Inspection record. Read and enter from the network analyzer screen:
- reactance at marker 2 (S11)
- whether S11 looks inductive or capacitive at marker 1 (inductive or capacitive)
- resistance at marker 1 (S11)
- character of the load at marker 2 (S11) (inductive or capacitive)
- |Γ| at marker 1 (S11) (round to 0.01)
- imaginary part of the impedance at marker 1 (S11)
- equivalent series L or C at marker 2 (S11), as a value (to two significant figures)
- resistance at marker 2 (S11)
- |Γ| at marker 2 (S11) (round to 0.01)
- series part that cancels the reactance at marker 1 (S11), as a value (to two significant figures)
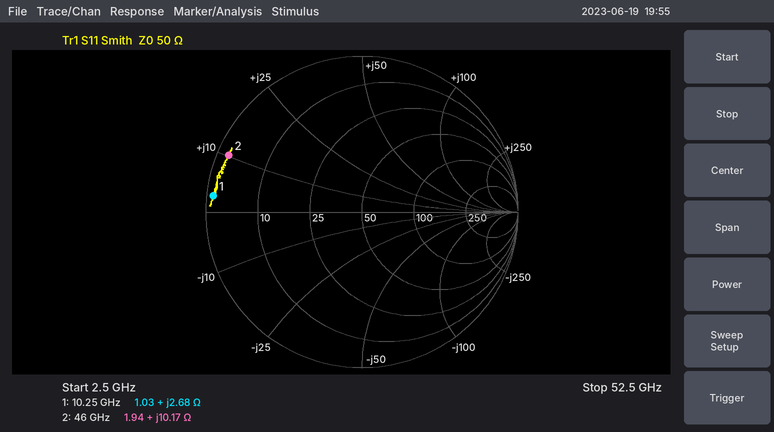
+10.17 Ω
inductive
1.03 Ω
inductive
0.96
+2.68 Ω
35 pH
1.94 Ω
0.93
5.8 pF
